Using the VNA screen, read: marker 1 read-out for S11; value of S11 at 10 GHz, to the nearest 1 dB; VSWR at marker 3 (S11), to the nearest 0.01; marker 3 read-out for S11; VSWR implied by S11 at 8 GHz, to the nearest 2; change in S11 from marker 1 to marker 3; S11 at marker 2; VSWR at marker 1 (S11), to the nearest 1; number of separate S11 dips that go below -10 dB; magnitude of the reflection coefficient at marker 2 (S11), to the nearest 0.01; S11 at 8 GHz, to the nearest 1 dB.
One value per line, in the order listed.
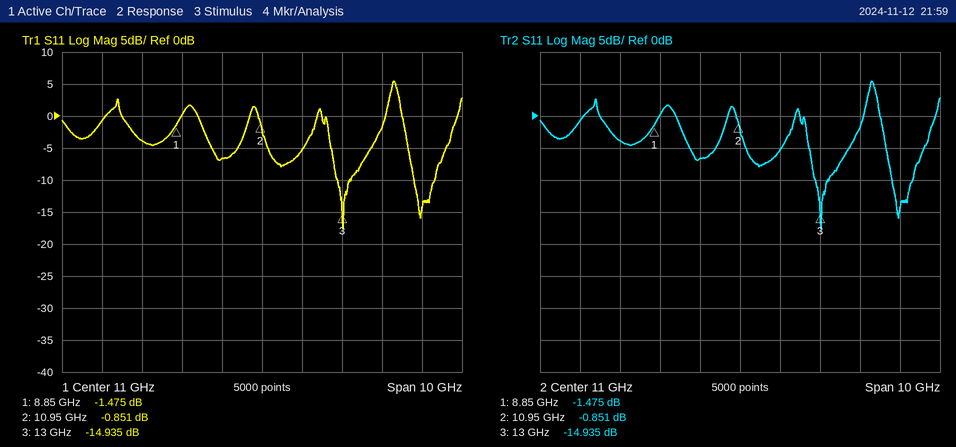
-1.475 dB
-7 dB
1.44
-14.935 dB
4
-13.460 dB
-0.851 dB
12
2
0.91
-4 dB
